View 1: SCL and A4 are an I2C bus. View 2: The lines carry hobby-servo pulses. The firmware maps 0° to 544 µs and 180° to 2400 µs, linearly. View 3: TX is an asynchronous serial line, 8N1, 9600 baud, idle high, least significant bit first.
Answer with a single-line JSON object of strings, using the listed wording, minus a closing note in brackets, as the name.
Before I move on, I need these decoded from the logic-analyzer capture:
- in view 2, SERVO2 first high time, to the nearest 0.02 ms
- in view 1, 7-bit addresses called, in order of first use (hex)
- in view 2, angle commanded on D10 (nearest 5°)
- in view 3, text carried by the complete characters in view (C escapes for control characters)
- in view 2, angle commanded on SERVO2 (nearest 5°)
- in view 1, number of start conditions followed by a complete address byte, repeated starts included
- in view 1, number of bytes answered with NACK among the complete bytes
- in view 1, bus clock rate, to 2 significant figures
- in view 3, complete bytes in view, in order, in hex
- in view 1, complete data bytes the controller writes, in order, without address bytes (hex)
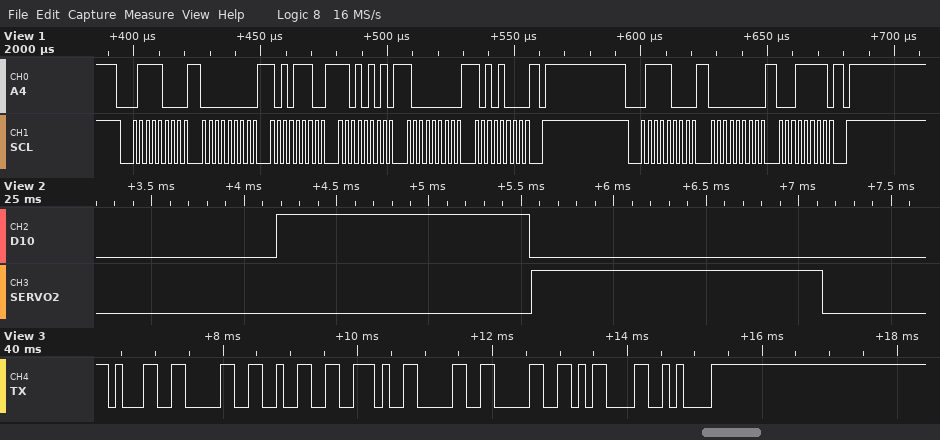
{"in view 2, SERVO2 first high time, to the nearest 0.02 ms": "1.58 ms", "in view 1, 7-bit addresses called, in order of first use": "0x3C", "in view 2, angle commanded on D10": "80°", "in view 3, text carried by the complete characters in view": "\"102.00\\r\\n\"", "in view 2, angle commanded on SERVO2": "100°", "in view 1, number of start conditions followed by a complete address byte, repeated starts included": "2", "in view 1, number of bytes answered with NACK among the complete bytes": "0", "in view 1, bus clock rate, to 2 significant figures": "400 kHz", "in view 3, complete bytes in view, in order, in hex": "0x31 0x30 0x32 0x2E 0x30 0x30 0x0D 0x0A", "in view 1, complete data bytes the controller writes, in order, without address bytes": "00 AE D5 80 A8 00 1F"}
